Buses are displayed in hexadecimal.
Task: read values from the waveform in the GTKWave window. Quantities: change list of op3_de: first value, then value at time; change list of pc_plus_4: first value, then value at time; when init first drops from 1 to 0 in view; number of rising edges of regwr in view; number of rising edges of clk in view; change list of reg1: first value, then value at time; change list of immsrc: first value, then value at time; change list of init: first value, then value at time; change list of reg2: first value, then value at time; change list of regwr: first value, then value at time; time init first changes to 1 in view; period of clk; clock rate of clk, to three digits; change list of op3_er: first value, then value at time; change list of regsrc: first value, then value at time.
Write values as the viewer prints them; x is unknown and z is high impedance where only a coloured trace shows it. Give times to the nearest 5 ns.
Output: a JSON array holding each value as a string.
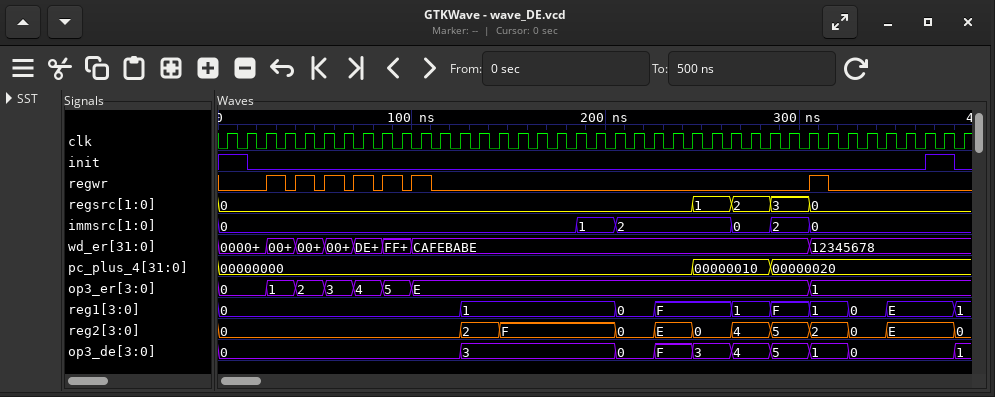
["0, 3 at 125 ns, 0 at 205 ns, F at 225 ns, 3 at 245 ns, 4 at 265 ns, 5 at 285 ns, 1 at 305 ns, 0 at 325 ns, 1 at 380 ns", "00000000, 00000010 at 245 ns, 00000020 at 285 ns", "15 ns", "7", "39", "0, 1 at 125 ns, 0 at 205 ns, F at 225 ns, 1 at 265 ns, F at 285 ns, 1 at 305 ns, 0 at 325 ns, E at 345 ns, 1 at 380 ns", "0, 1 at 185 ns, 2 at 205 ns, 0 at 265 ns, 2 at 285 ns, 0 at 305 ns", "1, 0 at 15 ns, 1 at 365 ns, 0 at 380 ns", "0, 2 at 125 ns, F at 145 ns, 0 at 205 ns, E at 225 ns, 0 at 245 ns, 4 at 265 ns, 5 at 285 ns, 2 at 305 ns, 0 at 325 ns, E at 345 ns, 0 at 380 ns", "0, 1 at 25 ns, 0 at 35 ns, 1 at 40 ns, 0 at 50 ns, 1 at 55 ns, 0 at 65 ns, 1 at 70 ns, 0 at 80 ns, 1 at 85 ns, 0 at 95 ns, 1 at 100 ns, 0 at 110 ns, 1 at 305 ns, 0 at 315 ns", "365 ns", "10 ns", "100 MHz", "0, 1 at 25 ns, 2 at 40 ns, 3 at 55 ns, 4 at 70 ns, 5 at 85 ns, E at 100 ns, 1 at 305 ns", "0, 1 at 245 ns, 2 at 265 ns, 3 at 285 ns, 0 at 305 ns"]
